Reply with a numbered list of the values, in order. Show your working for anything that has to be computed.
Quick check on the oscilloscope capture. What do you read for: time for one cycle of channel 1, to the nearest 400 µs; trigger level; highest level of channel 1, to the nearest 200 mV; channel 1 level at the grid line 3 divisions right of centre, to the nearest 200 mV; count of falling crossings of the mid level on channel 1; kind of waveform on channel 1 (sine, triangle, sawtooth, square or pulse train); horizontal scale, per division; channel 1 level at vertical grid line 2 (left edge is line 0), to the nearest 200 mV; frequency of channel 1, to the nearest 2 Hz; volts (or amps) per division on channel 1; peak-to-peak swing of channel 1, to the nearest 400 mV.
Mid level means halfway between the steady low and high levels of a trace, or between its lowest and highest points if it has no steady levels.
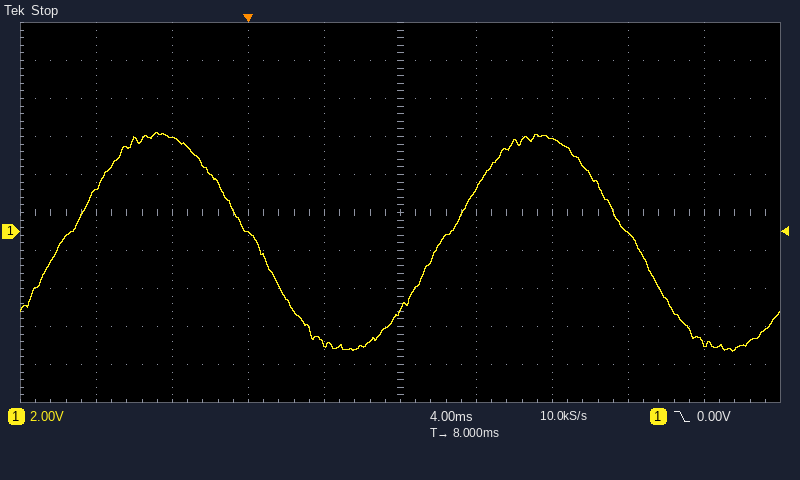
1. 20.0 ms
2. 0.00 V
3. 5.2 V
4. 0.0 V
5. 2
6. sine
7. 4 ms
8. 5.0 V
9. 1 / 20.0 ms ≈ 50 Hz
10. 2 V
11. 11.6 V
